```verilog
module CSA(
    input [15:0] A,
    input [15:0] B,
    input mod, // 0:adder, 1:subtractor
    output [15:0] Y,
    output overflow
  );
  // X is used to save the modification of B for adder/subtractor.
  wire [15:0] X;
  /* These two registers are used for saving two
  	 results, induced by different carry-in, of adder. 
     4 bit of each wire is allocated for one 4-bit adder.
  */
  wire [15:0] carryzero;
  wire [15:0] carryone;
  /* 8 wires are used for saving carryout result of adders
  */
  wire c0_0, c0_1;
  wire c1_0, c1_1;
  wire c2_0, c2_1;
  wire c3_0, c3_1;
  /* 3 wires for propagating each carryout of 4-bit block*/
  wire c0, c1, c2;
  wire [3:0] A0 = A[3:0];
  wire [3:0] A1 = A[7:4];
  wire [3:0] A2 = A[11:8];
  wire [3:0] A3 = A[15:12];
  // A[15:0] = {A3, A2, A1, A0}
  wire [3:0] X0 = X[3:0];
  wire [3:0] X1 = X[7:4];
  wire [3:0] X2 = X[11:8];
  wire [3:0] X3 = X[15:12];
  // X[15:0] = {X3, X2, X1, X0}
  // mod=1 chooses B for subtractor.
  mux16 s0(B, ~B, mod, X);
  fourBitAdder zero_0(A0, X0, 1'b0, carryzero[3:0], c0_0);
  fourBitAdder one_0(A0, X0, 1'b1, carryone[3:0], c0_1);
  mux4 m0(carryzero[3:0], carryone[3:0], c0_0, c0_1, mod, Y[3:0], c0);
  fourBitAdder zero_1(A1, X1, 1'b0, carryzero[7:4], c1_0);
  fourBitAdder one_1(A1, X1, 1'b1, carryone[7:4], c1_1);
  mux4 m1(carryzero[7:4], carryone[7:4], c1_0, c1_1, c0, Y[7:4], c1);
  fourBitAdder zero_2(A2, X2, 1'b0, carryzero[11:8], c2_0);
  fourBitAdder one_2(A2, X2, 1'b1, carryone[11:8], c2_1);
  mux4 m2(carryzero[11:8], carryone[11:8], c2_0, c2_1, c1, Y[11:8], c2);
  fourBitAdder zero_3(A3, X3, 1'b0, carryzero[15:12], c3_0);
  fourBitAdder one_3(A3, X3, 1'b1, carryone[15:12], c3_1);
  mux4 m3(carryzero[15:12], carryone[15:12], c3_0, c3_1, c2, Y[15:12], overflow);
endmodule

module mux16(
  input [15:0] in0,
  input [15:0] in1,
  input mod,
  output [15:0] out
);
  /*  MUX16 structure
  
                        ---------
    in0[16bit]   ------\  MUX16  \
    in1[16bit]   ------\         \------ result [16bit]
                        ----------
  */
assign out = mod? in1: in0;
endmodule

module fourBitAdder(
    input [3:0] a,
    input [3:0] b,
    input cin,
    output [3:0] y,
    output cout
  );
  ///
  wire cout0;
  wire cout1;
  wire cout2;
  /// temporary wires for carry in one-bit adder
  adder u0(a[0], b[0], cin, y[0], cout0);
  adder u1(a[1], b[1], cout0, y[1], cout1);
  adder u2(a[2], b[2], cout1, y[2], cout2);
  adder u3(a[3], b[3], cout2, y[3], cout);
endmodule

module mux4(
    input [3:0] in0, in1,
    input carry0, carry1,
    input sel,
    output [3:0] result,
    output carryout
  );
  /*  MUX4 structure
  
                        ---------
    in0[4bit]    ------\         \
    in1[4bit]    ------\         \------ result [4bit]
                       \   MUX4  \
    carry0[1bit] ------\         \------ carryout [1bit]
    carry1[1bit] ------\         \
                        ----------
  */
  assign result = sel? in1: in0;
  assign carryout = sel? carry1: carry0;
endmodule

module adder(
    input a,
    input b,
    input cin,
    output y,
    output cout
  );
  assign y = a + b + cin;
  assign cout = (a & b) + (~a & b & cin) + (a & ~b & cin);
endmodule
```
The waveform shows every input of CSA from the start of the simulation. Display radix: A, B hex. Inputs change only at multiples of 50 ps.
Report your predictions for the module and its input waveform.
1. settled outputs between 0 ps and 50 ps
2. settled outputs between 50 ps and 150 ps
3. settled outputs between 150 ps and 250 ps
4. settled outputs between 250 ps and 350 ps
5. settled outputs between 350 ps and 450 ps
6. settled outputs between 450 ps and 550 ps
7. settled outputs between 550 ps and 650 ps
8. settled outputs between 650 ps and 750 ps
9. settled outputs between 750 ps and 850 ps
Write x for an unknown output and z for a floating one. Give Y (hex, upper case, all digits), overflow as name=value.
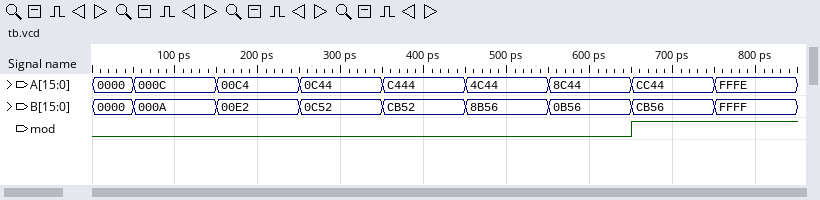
Y=0000, overflow=0
Y=0016, overflow=0
Y=01A6, overflow=0
Y=1896, overflow=0
Y=8F96, overflow=1
Y=D79A, overflow=0
Y=979A, overflow=0
Y=00EE, overflow=1
Y=FFFF, overflow=0
